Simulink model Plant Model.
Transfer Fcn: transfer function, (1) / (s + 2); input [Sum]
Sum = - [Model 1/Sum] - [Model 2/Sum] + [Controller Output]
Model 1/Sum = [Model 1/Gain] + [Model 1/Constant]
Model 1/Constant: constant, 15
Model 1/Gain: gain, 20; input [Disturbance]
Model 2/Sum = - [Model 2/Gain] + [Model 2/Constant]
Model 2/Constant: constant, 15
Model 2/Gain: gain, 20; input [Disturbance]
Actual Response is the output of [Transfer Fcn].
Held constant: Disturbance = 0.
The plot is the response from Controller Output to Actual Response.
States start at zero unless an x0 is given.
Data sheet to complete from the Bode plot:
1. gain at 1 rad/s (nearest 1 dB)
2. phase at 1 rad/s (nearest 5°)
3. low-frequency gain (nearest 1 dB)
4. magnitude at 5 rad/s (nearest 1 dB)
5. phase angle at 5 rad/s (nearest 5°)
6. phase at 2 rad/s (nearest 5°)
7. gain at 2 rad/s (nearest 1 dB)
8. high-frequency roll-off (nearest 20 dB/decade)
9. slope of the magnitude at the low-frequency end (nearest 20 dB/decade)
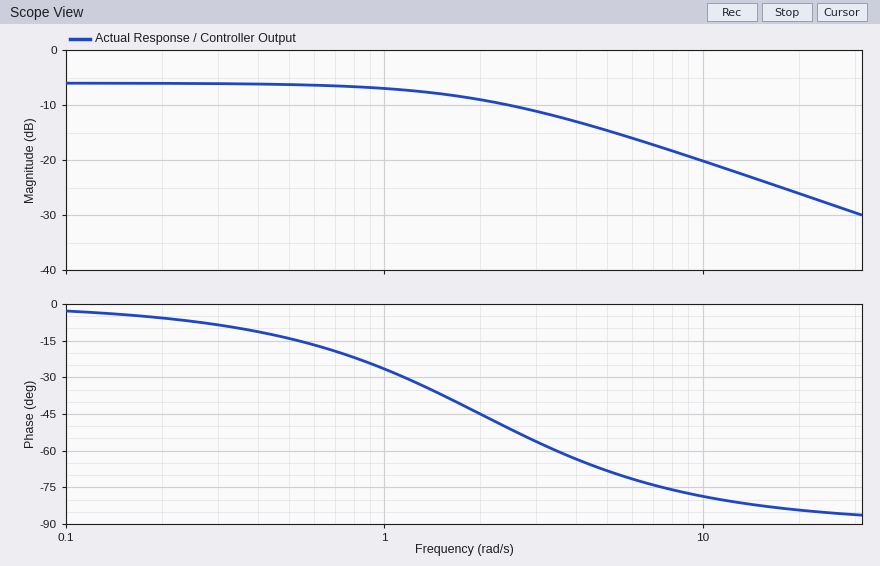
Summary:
-7 dB
-25°
-6 dB
-15 dB
-70°
-45°
-9 dB
-20 dB/decade
0 dB/decade
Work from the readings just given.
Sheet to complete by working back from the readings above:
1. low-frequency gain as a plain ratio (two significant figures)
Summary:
0.50
